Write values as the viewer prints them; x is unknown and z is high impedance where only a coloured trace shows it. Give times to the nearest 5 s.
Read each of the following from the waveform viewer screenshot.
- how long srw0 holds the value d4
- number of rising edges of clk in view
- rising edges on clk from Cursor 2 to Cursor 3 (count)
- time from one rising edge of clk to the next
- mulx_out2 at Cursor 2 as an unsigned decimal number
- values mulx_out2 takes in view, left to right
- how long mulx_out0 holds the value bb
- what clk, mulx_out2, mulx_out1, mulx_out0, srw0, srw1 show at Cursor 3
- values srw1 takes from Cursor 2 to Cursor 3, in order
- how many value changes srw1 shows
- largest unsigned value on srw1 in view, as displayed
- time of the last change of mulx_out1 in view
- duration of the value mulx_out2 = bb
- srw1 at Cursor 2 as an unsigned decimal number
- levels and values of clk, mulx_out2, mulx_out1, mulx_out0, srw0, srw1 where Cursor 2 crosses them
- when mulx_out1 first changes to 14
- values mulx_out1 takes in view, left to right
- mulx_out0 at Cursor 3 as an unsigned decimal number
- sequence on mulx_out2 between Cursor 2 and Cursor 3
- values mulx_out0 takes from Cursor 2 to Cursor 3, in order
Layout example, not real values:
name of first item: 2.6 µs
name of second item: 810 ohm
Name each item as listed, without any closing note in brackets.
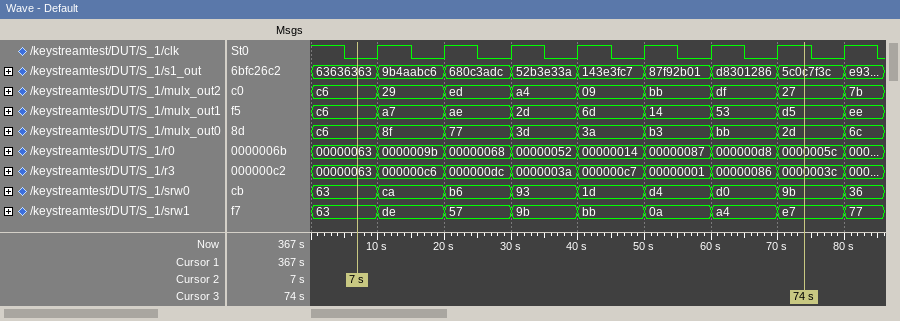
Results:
how long srw0 holds the value d4: 10 s
number of rising edges of clk in view: 8
rising edges on clk from Cursor 2 to Cursor 3: 7
time from one rising edge of clk to the next: 10 s
mulx_out2 at Cursor 2 as an unsigned decimal number: 198
values mulx_out2 takes in view, left to right: c6, 29, ed, a4, 09, bb, df, 27, 7b
how long mulx_out0 holds the value bb: 10 s
what clk, mulx_out2, mulx_out1, mulx_out0, srw0, srw1 show at Cursor 3: clk=1, mulx_out2=27, mulx_out1=d5, mulx_out0=2d, srw0=9b, srw1=e7
values srw1 takes from Cursor 2 to Cursor 3, in order: 63, de, 57, 9b, bb, 0a, a4, e7
how many value changes srw1 shows: 8
largest unsigned value on srw1 in view, as displayed: e7
time of the last change of mulx_out1 in view: 80 s
duration of the value mulx_out2 = bb: 10 s
srw1 at Cursor 2 as an unsigned decimal number: 99
levels and values of clk, mulx_out2, mulx_out1, mulx_out0, srw0, srw1 where Cursor 2 crosses them: clk=0, mulx_out2=c6, mulx_out1=c6, mulx_out0=c6, srw0=63, srw1=63
when mulx_out1 first changes to 14: 50 s
values mulx_out1 takes in view, left to right: c6, a7, ae, 2d, 6d, 14, 53, d5, ee
mulx_out0 at Cursor 3 as an unsigned decimal number: 45
sequence on mulx_out2 between Cursor 2 and Cursor 3: c6, 29, ed, a4, 09, bb, df, 27
values mulx_out0 takes from Cursor 2 to Cursor 3, in order: c6, 8f, 77, 3d, 3a, b3, bb, 2d
